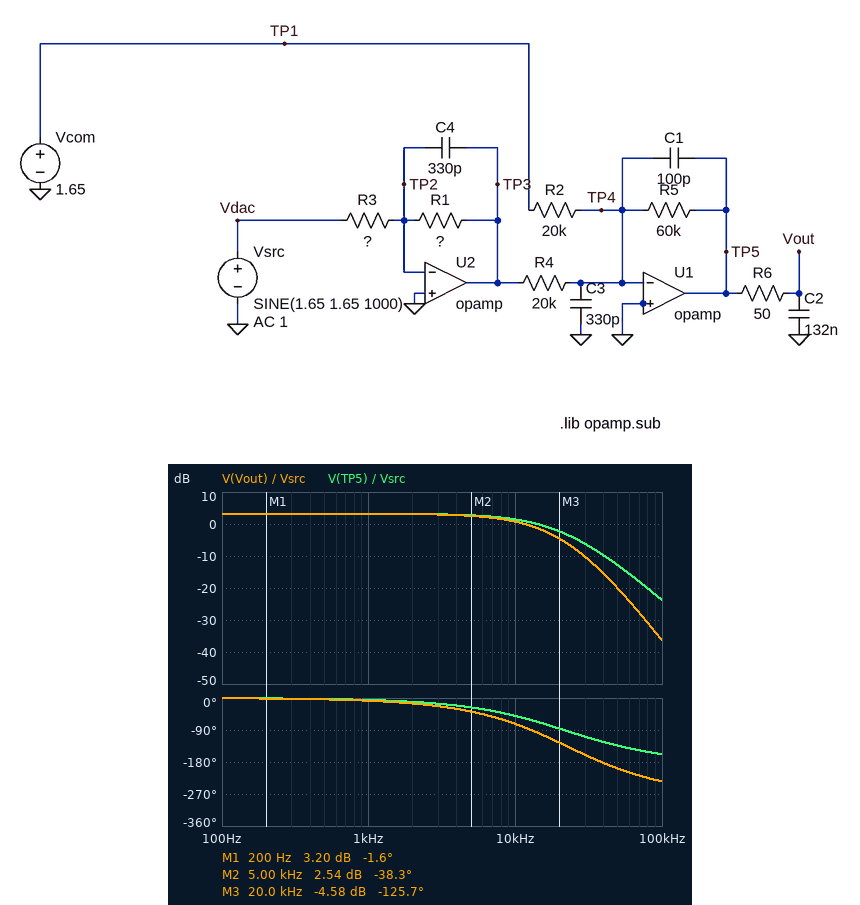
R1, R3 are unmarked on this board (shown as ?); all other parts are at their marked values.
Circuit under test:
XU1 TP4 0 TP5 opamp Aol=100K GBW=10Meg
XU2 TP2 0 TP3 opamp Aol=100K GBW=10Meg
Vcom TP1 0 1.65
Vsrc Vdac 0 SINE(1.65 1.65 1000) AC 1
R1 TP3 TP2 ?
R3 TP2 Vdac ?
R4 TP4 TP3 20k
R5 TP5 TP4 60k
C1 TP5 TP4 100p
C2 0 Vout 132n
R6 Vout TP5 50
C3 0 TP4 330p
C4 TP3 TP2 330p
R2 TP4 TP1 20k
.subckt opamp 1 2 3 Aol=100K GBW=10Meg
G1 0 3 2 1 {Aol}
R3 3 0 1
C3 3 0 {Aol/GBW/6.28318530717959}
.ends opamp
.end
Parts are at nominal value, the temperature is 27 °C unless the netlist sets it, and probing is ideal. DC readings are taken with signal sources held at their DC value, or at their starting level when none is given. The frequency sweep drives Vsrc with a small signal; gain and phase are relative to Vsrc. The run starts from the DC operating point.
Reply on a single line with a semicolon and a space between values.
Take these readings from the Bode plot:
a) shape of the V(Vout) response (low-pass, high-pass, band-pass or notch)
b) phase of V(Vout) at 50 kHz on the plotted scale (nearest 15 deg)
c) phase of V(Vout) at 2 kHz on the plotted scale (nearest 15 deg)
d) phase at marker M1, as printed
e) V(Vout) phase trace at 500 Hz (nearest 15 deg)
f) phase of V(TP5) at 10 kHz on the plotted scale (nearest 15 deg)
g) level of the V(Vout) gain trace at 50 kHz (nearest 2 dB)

low-pass; -195 deg; -15 deg; -1.6 deg; 0 deg; -45 deg; -20 dB
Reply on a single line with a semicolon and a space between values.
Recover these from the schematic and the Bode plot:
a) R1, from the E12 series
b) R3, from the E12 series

27 kΩ; 56 kΩ
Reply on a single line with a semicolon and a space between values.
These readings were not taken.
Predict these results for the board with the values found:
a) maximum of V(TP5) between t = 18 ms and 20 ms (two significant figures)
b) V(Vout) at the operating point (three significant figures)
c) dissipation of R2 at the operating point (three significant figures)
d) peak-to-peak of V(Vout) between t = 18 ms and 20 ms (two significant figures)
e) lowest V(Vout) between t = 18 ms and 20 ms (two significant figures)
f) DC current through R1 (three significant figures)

-180 mV; -2.56 V; 136 µW; 4.8 V; -4.9 V; 29.5 µA
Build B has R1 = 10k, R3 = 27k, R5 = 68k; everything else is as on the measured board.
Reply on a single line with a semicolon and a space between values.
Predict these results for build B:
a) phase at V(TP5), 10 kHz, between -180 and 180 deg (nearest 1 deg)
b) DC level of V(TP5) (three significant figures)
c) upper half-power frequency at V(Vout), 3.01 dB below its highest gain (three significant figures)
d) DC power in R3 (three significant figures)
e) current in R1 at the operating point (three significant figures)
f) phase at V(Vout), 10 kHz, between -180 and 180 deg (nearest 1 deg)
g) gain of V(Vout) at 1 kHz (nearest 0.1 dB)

-35 deg; -3.53 V; 14.1 kHz; 101 µW; 61.1 µA; -58 deg; 2.0 dB
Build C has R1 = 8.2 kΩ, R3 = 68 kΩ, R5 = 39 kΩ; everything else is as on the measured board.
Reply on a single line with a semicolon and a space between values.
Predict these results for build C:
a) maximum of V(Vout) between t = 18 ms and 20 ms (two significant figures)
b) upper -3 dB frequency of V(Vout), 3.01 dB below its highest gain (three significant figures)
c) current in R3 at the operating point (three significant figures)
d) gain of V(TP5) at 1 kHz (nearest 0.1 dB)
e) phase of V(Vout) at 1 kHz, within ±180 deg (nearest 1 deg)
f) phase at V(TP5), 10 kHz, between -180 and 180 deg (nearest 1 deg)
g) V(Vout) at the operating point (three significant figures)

-2.4 V; 17.7 kHz; 24.3 µA; -12.6 dB; -5 deg; -24 deg; -2.83 V
